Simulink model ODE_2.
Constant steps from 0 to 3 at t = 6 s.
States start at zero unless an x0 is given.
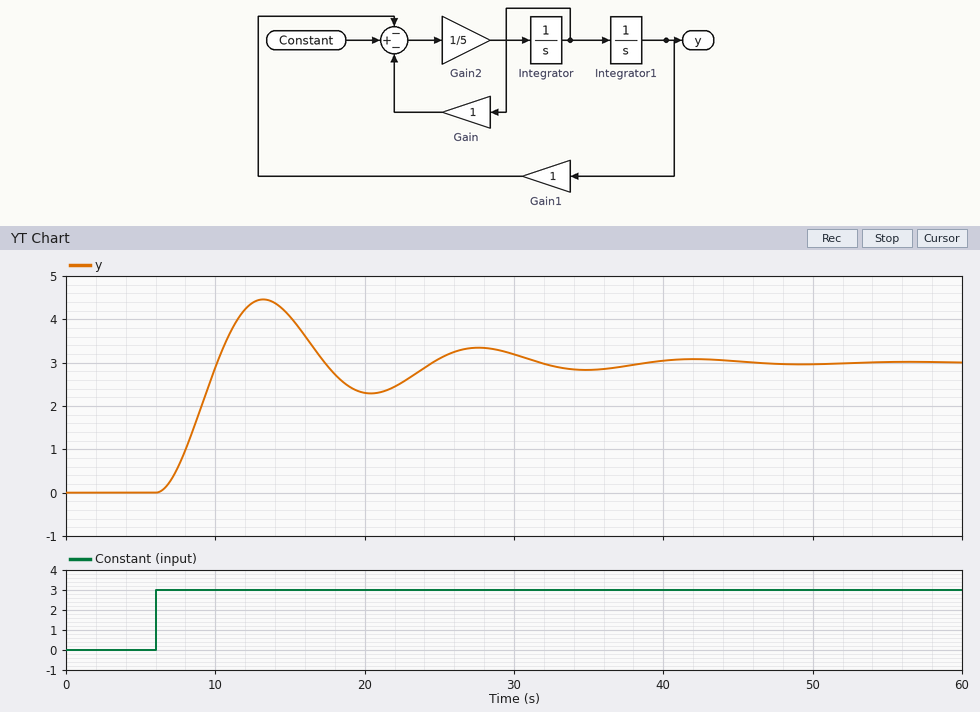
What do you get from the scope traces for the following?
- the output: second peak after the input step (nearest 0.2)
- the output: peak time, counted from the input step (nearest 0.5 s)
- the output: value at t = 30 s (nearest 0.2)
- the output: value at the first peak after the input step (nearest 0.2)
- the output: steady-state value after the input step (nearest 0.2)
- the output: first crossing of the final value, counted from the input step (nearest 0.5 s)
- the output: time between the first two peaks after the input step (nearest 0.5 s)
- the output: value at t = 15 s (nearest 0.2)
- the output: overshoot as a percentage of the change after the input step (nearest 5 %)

3.4
7.0 s
3.2
4.4
3.0
4.0 s
14.5 s
4.0
50 %
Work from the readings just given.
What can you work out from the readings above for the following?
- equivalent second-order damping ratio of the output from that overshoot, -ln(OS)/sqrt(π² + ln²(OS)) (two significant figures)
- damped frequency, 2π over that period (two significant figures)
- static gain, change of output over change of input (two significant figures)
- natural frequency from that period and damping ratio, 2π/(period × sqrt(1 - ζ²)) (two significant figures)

0.22
0.43 rad/s
1.0
0.44 rad/s
